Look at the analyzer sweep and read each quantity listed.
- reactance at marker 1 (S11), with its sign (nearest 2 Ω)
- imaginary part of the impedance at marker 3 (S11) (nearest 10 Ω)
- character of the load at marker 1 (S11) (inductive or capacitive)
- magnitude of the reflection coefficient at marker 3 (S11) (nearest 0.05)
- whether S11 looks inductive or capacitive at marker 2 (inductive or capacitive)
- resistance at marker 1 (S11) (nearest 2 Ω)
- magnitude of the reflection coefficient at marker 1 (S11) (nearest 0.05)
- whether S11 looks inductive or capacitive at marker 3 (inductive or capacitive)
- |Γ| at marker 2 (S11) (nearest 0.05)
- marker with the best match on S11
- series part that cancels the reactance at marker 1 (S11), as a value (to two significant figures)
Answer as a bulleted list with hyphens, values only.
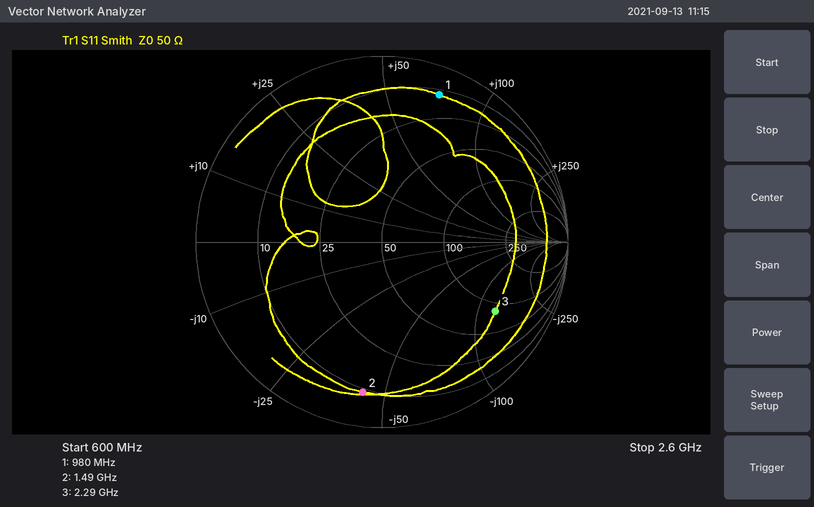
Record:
- +72 Ω
- -130 Ω
- inductive
- 0.70
- capacitive
- 12 Ω
- 0.85
- capacitive
- 0.80
- marker 3
- 2.3 pF
